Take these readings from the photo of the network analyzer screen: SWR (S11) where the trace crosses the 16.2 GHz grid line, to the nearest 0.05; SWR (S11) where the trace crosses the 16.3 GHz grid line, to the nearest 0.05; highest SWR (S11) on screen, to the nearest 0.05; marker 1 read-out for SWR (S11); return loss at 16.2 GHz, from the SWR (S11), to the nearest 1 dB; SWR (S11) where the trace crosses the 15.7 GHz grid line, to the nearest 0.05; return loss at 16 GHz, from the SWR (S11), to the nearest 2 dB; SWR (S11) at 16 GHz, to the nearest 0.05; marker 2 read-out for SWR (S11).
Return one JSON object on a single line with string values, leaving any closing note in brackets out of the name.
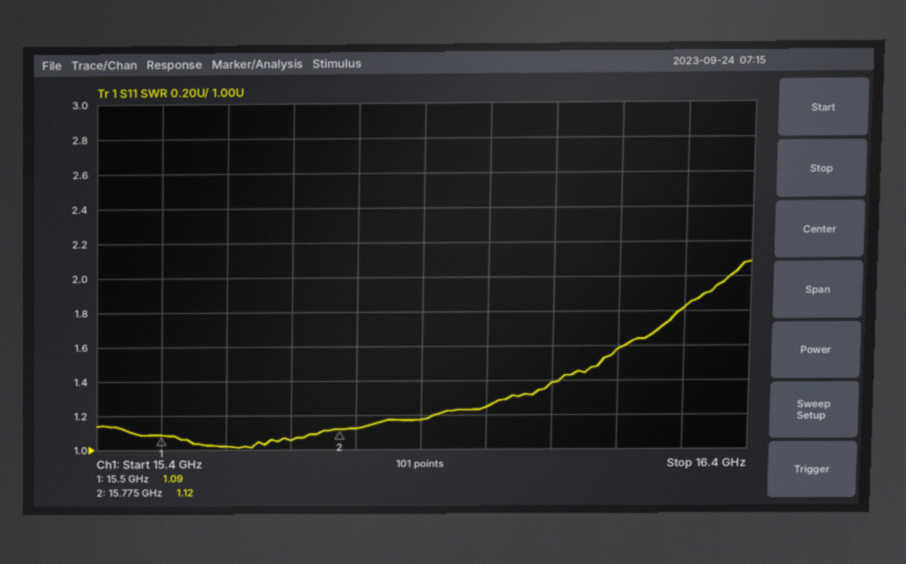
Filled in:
{"SWR (S11) where the trace crosses the 16.2 GHz grid line, to the nearest 0.05": "1.60", "SWR (S11) where the trace crosses the 16.3 GHz grid line, to the nearest 0.05": "1.80", "highest SWR (S11) on screen, to the nearest 0.05": "2.10", "marker 1 read-out for SWR": "1.09", "return loss at 16.2 GHz, from the SWR (S11), to the nearest 1 dB": "13 dB", "SWR (S11) where the trace crosses the 15.7 GHz grid line, to the nearest 0.05": "1.05", "return loss at 16 GHz, from the SWR (S11), to the nearest 2 dB": "20 dB", "SWR (S11) at 16 GHz, to the nearest 0.05": "1.25", "marker 2 read-out for SWR": "1.12"}
